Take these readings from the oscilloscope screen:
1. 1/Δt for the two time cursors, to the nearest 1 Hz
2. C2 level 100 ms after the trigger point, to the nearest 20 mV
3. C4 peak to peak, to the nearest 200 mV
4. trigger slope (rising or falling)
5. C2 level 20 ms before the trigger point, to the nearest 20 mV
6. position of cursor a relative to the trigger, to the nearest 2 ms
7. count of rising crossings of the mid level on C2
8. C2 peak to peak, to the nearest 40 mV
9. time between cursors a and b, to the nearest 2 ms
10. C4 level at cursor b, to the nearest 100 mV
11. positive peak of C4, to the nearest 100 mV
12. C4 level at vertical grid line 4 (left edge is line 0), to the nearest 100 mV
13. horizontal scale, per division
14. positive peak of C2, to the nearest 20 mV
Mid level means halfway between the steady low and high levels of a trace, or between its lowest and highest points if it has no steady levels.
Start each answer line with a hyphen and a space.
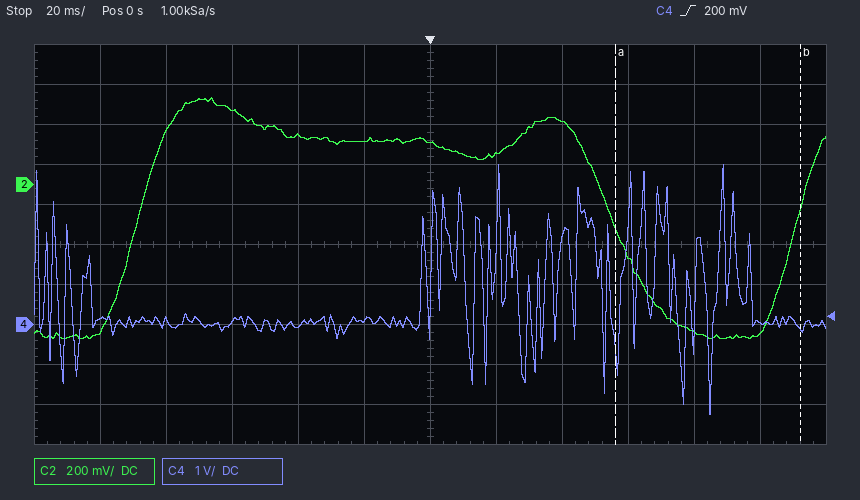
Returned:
- 18 Hz
- -740 mV
- 6.2 V
- rising
- 220 mV
- +56 ms
- 2
- 1.20 V
- 56 ms
- -100 mV
- 4.0 V
- 0.0 V
- 20 ms
- 440 mV
